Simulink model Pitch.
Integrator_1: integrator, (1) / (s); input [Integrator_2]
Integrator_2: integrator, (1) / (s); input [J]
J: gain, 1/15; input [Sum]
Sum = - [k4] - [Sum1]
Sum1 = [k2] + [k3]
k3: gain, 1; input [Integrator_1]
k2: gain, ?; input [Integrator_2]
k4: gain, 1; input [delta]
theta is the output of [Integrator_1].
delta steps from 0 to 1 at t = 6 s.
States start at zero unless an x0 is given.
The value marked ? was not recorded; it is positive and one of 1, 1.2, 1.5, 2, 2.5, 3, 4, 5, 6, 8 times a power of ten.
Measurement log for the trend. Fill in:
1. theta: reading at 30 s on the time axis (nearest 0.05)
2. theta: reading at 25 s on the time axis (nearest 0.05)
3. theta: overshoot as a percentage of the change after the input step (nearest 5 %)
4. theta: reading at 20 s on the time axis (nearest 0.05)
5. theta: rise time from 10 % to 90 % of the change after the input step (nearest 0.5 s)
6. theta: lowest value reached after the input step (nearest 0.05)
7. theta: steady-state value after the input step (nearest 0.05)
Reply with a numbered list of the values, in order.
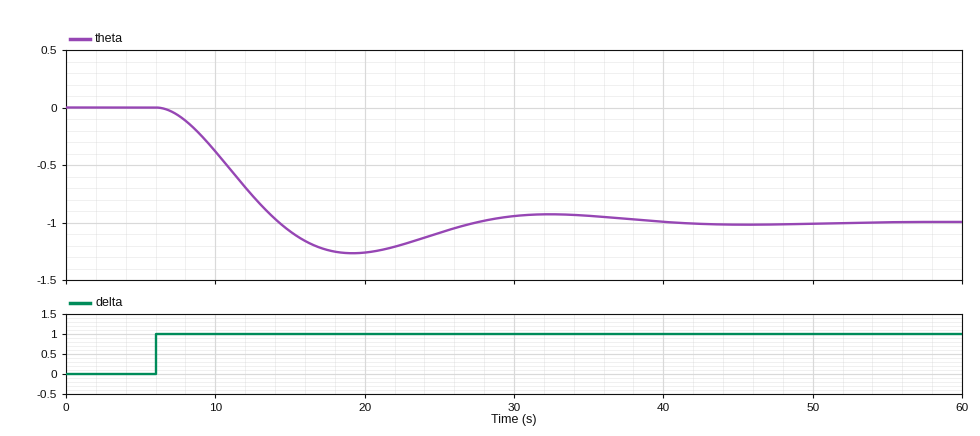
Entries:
1. -0.95
2. -1.10
3. 25 %
4. -1.25
5. 5.5 s
6. -1.25
7. -1.00
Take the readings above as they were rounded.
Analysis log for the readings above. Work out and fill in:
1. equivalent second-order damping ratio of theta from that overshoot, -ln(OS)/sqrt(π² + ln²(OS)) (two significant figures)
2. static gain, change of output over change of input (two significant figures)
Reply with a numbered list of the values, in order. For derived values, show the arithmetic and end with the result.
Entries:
1. ln(0.25) = -1.386; 1.386 / sqrt(9.870 + 1.922) = 0.40
2. (-1 - 0) / (1 - 0) = -1.0
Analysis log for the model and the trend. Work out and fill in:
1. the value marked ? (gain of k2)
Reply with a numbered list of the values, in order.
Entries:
1. 3
